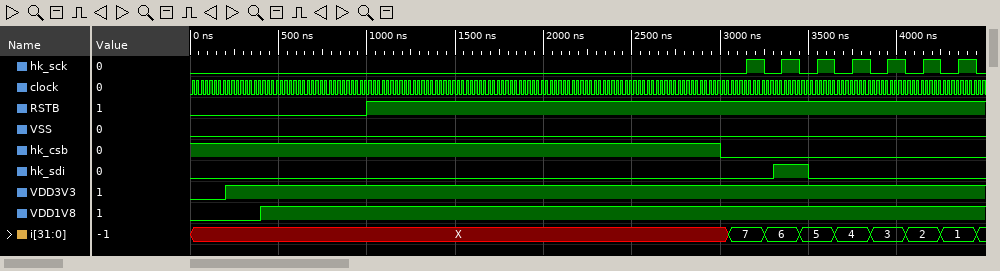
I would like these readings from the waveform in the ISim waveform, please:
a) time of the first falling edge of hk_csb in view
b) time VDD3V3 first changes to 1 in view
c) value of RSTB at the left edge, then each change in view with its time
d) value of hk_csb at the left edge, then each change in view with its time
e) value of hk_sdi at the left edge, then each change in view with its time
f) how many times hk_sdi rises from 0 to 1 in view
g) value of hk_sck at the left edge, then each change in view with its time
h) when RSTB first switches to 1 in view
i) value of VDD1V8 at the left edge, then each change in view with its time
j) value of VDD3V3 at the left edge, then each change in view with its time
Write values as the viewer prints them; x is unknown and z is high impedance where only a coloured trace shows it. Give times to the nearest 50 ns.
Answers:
3000 ns
200 ns
0, 1 at 1000 ns
1, 0 at 3000 ns
0, 1 at 3300 ns, 0 at 3500 ns
1
0, 1 at 3150 ns, 0 at 3250 ns, 1 at 3350 ns, 0 at 3450 ns, 1 at 3550 ns, 0 at 3650 ns, 1 at 3750 ns, 0 at 3850 ns, 1 at 3950 ns, 0 at 4050 ns, 1 at 4150 ns, 0 at 4250 ns, 1 at 4350 ns, 0 at 4450 ns
1000 ns
0, 1 at 400 ns
0, 1 at 200 ns
